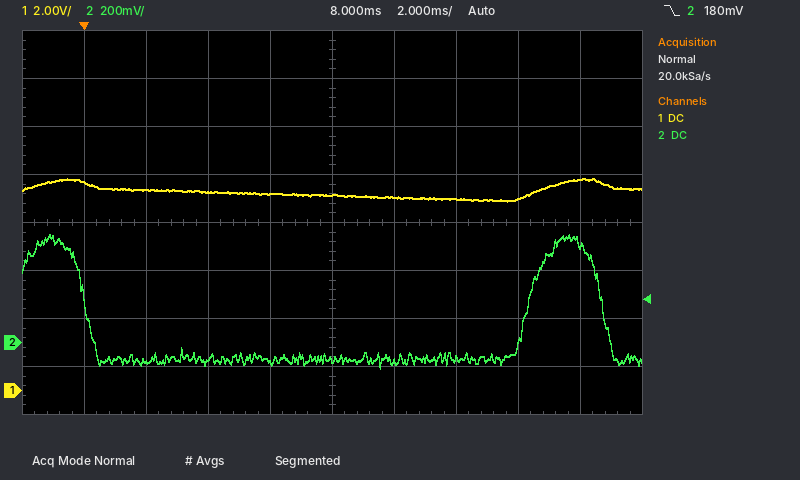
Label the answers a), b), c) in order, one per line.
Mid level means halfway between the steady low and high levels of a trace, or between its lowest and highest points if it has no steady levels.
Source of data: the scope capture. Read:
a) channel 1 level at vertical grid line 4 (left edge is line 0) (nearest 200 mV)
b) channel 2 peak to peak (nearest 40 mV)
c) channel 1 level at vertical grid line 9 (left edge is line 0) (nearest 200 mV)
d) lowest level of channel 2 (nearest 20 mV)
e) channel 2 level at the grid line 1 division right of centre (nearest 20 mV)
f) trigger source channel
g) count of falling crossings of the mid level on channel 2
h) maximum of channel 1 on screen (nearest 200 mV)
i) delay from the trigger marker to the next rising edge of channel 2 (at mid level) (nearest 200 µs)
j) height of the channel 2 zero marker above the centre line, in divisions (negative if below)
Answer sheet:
a) 8.2 V
b) 560 mV
c) 8.8 V
d) -100 mV
e) -80 mV
f) channel 2
g) 2
h) 8.8 V
i) 14.4 ms
j) -2.5 div
